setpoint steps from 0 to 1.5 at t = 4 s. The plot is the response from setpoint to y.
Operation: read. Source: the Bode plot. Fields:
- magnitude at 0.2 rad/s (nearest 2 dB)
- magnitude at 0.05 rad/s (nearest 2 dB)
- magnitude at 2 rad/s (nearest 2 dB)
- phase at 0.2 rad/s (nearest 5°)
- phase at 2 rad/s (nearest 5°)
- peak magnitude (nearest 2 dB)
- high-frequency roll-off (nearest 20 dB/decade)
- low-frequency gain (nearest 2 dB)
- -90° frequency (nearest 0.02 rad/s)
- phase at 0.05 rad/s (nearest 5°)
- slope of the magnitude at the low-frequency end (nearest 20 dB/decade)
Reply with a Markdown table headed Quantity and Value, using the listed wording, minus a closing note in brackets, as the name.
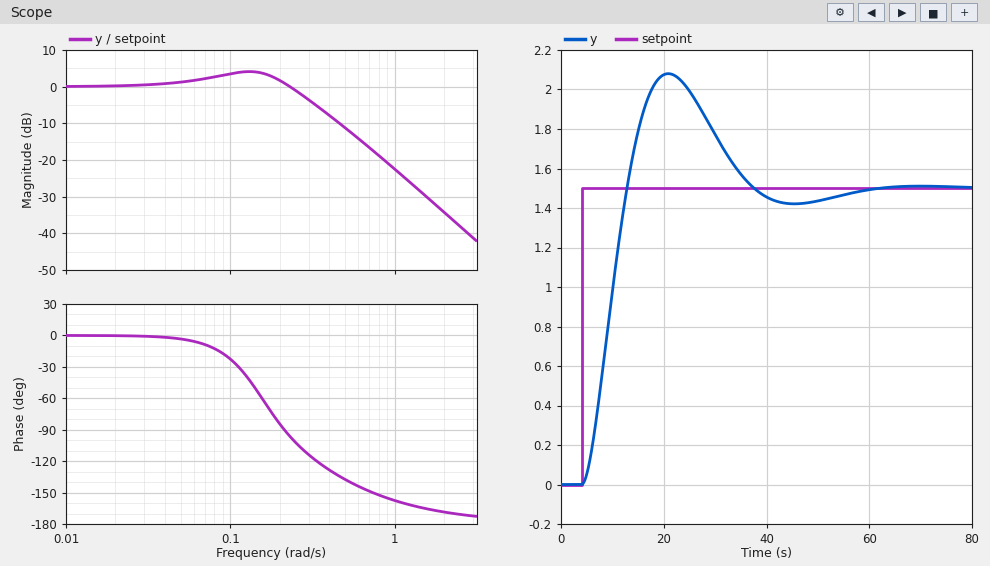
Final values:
| Quantity | Value |
|---|---|
| magnitude at 0.2 rad/s | 2 dB |
| magnitude at 0.05 rad/s | 2 dB |
| magnitude at 2 rad/s | -34 dB |
| phase at 0.2 rad/s | -85° |
| phase at 2 rad/s | -170° |
| peak magnitude | 4 dB |
| high-frequency roll-off | -40 dB/decade |
| low-frequency gain | 0 dB |
| -90° frequency | 0.22 rad/s |
| phase at 0.05 rad/s | -5° |
| slope of the magnitude at the low-frequency end | 0 dB/decade |
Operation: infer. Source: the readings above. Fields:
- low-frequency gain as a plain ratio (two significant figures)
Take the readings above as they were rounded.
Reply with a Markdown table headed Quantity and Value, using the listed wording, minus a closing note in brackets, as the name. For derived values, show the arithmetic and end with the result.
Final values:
| Quantity | Value |
|---|---|
| low-frequency gain as a plain ratio | 10^(0 / 20) = 1.0 |
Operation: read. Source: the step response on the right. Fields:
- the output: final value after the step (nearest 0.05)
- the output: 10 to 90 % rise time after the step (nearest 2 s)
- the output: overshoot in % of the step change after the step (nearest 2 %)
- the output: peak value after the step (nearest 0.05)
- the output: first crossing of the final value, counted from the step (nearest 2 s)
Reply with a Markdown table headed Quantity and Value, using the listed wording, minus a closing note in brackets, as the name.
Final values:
| Quantity | Value |
|---|---|
| the output: final value after the step | 1.50 |
| the output: 10 to 90 % rise time after the step | 6 s |
| the output: overshoot in % of the step change after the step | 38 % |
| the output: peak value after the step | 2.10 |
| the output: first crossing of the final value, counted from the step | 8 s |
